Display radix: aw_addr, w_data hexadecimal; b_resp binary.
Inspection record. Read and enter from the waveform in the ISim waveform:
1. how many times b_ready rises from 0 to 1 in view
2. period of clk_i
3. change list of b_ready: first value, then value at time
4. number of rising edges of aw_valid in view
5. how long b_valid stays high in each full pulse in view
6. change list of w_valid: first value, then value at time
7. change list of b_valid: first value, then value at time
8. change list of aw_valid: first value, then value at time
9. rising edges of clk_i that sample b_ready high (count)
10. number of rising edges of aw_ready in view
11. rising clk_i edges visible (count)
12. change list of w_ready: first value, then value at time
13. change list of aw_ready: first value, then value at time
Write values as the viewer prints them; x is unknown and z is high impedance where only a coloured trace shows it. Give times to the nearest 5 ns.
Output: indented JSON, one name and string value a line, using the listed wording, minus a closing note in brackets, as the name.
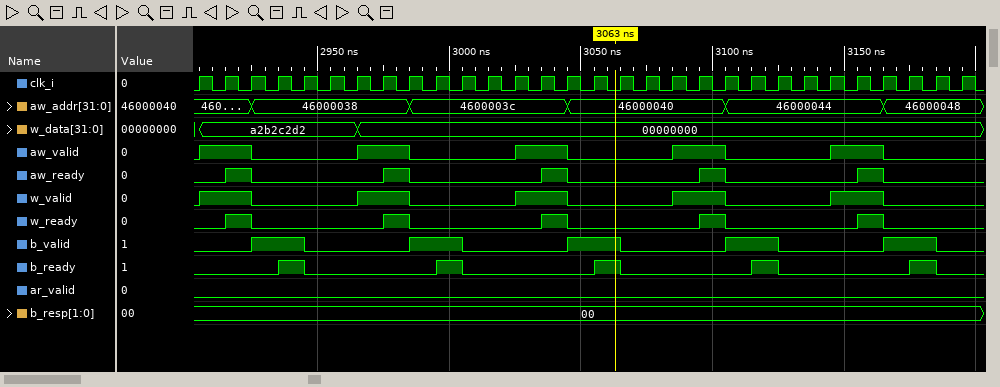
{
  "how many times b_ready rises from 0 to 1 in view": "5",
  "period of clk_i": "10 ns",
  "change list of b_ready: first value, then value at time": "0, 1 at 2935 ns, 0 at 2945 ns, 1 at 2995 ns, 0 at 3005 ns, 1 at 3055 ns, 0 at 3065 ns, 1 at 3115 ns, 0 at 3125 ns, 1 at 3175 ns, 0 at 3185 ns",
  "number of rising edges of aw_valid in view": "5",
  "how long b_valid stays high in each full pulse in view": "20 ns, 20 ns, 20 ns, 20 ns, 20 ns",
  "change list of w_valid: first value, then value at time": "0, 1 at 2905 ns, 0 at 2925 ns, 1 at 2965 ns, 0 at 2985 ns, 1 at 3025 ns, 0 at 3045 ns, 1 at 3085 ns, 0 at 3105 ns, 1 at 3145 ns, 0 at 3165 ns",
  "change list of b_valid: first value, then value at time": "0, 1 at 2925 ns, 0 at 2945 ns, 1 at 2985 ns, 0 at 3005 ns, 1 at 3045 ns, 0 at 3065 ns, 1 at 3105 ns, 0 at 3125 ns, 1 at 3165 ns, 0 at 3185 ns",
  "change list of aw_valid: first value, then value at time": "0, 1 at 2905 ns, 0 at 2925 ns, 1 at 2965 ns, 0 at 2985 ns, 1 at 3025 ns, 0 at 3045 ns, 1 at 3085 ns, 0 at 3105 ns, 1 at 3145 ns, 0 at 3165 ns",
  "rising edges of clk_i that sample b_ready high": "5",
  "number of rising edges of aw_ready in view": "5",
  "rising clk_i edges visible": "30",
  "change list of w_ready: first value, then value at time": "0, 1 at 2915 ns, 0 at 2925 ns, 1 at 2975 ns, 0 at 2985 ns, 1 at 3035 ns, 0 at 3045 ns, 1 at 3095 ns, 0 at 3105 ns, 1 at 3155 ns, 0 at 3165 ns",
  "change list of aw_ready: first value, then value at time": "0, 1 at 2915 ns, 0 at 2925 ns, 1 at 2975 ns, 0 at 2985 ns, 1 at 3035 ns, 0 at 3045 ns, 1 at 3095 ns, 0 at 3105 ns, 1 at 3155 ns, 0 at 3165 ns"
}
